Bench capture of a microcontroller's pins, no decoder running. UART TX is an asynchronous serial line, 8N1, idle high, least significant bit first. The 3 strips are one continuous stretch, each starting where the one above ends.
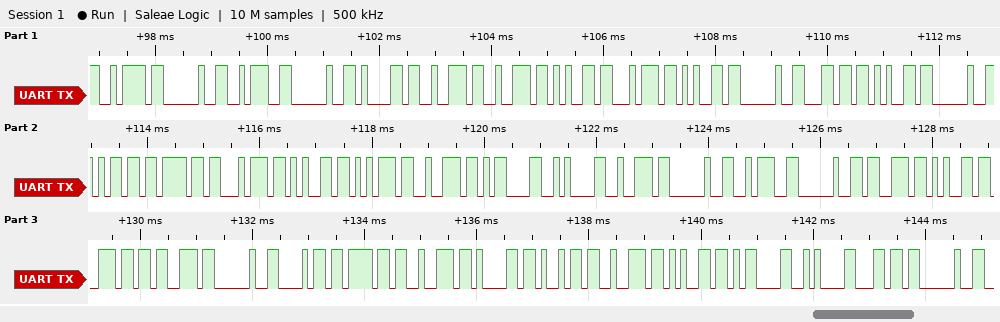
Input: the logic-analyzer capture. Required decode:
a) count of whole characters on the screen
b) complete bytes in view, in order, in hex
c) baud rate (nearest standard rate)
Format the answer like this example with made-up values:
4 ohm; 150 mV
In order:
42; 7A 20 3A 20 61 72 72 65 74 65 20 6C 65 20 6D 6F 74 65 75 72 0D 0A 72 20 3A 20 73 65 6E 73 20 68 6F 72 61 69 72 65 0D 0A 6C 20; 9600 baud
